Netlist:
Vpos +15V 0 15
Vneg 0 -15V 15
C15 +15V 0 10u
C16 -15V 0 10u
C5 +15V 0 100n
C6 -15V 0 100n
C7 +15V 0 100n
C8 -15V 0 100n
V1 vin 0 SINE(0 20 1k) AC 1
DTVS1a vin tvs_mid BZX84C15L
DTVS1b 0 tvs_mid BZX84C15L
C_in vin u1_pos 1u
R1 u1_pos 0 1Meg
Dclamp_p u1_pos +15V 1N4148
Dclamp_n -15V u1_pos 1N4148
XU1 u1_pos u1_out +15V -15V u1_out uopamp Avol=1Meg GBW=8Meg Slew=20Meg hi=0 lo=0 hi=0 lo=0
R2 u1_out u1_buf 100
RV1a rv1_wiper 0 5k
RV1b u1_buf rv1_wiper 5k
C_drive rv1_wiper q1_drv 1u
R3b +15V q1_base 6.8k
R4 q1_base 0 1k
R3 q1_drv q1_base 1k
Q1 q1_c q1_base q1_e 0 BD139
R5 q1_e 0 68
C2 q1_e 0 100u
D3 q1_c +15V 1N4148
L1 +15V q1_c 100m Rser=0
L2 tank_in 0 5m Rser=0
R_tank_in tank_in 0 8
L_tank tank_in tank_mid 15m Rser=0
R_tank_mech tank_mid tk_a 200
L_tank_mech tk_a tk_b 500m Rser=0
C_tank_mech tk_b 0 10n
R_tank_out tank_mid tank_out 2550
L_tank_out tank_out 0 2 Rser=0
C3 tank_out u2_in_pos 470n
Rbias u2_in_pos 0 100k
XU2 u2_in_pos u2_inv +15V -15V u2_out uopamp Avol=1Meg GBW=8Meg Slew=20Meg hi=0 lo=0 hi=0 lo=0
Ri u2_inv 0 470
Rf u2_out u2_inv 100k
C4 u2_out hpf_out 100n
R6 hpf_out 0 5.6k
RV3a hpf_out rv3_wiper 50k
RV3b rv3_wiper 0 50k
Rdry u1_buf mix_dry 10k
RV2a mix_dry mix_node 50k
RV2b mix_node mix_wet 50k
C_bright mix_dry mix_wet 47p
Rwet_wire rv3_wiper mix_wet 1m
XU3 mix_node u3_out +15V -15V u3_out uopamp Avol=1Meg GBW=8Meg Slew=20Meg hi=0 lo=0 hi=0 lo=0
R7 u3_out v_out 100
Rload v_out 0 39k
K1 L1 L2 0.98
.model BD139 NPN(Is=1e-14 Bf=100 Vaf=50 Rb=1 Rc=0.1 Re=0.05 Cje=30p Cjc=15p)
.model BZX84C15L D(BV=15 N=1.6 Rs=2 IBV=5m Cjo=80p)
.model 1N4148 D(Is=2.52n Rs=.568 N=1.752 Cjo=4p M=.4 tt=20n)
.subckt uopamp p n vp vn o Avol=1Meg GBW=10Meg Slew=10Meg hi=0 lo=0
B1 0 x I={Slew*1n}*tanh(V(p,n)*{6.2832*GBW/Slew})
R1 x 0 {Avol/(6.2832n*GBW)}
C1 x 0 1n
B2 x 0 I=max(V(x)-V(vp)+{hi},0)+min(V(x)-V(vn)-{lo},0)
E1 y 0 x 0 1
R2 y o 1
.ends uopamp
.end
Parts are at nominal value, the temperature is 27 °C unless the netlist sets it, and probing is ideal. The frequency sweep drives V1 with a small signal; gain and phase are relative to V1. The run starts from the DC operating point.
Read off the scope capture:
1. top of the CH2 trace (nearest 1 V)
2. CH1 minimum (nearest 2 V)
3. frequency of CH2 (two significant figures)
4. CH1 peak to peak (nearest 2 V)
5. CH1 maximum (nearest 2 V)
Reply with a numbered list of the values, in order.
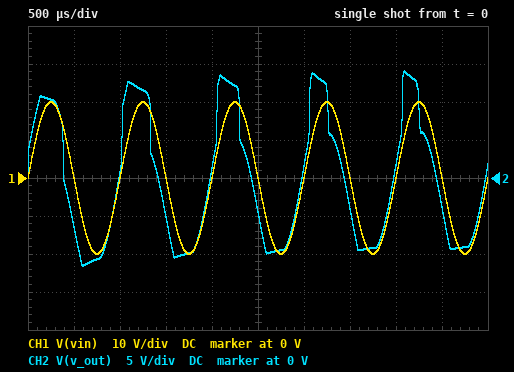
1. 14 V
2. -20 V
3. 1.0 kHz
4. 40 V
5. 20 V
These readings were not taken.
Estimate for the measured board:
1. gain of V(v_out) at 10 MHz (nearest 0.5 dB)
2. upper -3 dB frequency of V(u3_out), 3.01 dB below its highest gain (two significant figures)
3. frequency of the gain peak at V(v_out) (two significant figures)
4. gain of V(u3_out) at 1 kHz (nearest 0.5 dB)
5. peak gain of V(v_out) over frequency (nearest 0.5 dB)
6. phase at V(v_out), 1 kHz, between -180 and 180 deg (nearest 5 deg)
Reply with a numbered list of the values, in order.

1. -11.5 dB
2. 2.2 kHz
3. 2.2 kHz
4. 26.0 dB
5. 31.0 dB
6. 55 deg
